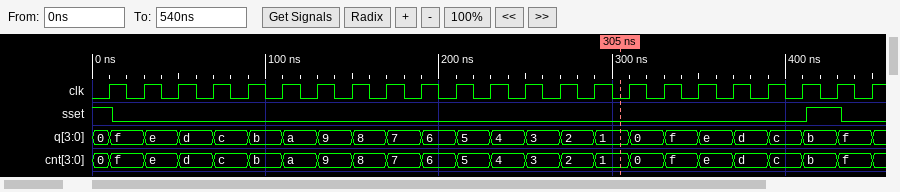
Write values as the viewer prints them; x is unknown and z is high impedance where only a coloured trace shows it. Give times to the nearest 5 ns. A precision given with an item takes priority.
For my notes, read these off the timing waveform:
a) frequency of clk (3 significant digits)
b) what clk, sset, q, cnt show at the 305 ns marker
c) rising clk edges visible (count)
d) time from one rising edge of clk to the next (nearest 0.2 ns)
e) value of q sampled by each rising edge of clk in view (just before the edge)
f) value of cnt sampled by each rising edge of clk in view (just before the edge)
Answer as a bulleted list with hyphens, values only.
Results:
- 50.0 MHz
- clk=0, sset=0, q=1, cnt=1
- 23
- 20 ns
- 0, f, e, d, c, b, a, 9, 8, 7, 6, 5, 4, 3, 2, 1, 0, f, e, d, c, b, f
- 0, f, e, d, c, b, a, 9, 8, 7, 6, 5, 4, 3, 2, 1, 0, f, e, d, c, b, f
